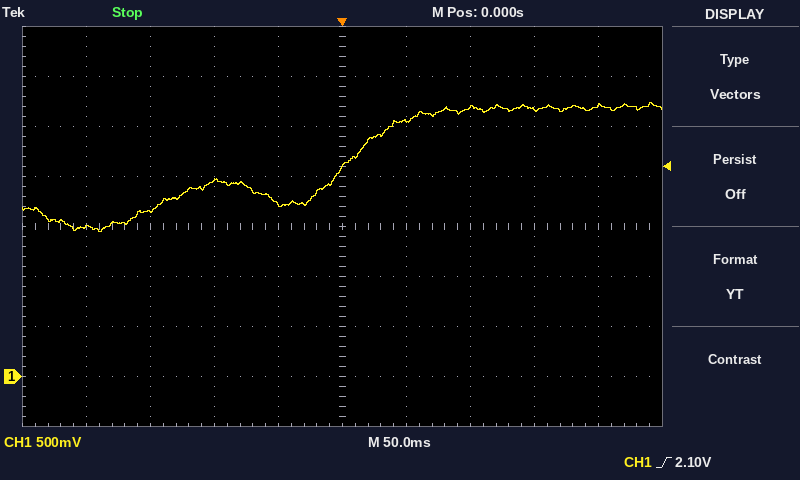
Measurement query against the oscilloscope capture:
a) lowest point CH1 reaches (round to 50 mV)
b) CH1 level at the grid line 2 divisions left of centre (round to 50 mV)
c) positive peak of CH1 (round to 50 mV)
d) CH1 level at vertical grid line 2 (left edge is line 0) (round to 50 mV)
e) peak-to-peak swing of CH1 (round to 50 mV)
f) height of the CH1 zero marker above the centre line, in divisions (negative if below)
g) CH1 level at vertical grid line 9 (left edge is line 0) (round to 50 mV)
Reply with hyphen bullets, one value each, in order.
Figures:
- 1.45 V
- 1.95 V
- 2.75 V
- 1.65 V
- 1.30 V
- -3.0 div
- 2.70 V
